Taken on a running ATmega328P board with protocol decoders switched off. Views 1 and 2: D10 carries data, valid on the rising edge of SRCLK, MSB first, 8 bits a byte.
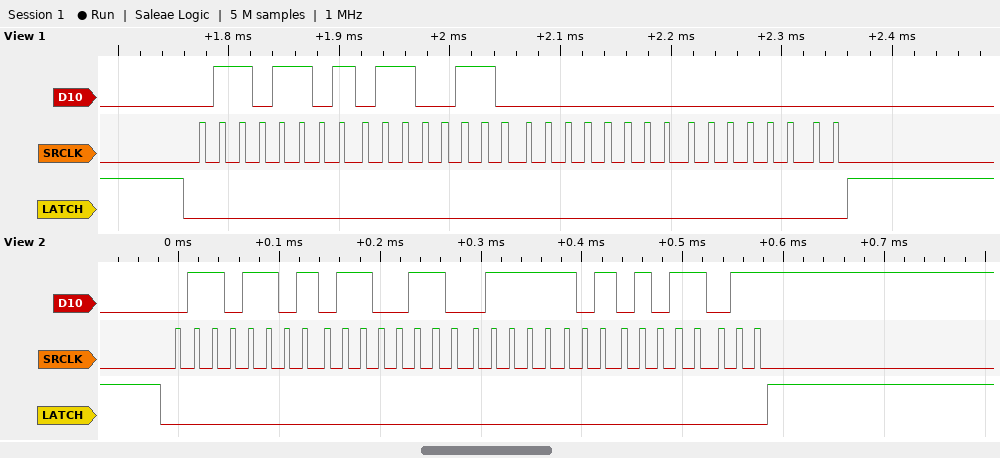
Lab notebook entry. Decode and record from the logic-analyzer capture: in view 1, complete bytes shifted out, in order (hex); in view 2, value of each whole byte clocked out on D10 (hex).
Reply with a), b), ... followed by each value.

a) 6D 66 00 00
b) 6D 66 7D 5B
